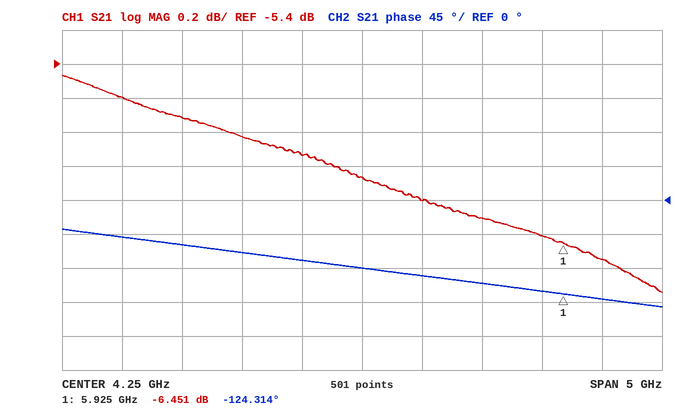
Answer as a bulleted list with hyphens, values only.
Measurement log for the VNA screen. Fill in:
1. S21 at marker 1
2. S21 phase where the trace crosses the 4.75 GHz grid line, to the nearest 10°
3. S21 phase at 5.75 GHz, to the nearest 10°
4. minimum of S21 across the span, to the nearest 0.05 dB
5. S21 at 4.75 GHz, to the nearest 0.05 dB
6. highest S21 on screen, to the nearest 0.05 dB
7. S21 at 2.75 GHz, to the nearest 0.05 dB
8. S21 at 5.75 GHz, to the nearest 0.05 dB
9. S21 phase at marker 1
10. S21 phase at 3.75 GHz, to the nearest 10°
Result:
- -6.451 dB
- -100°
- -120°
- -6.75 dB
- -6.20 dB
- -5.45 dB
- -5.70 dB
- -6.40 dB
- -124.314°
- -80°
